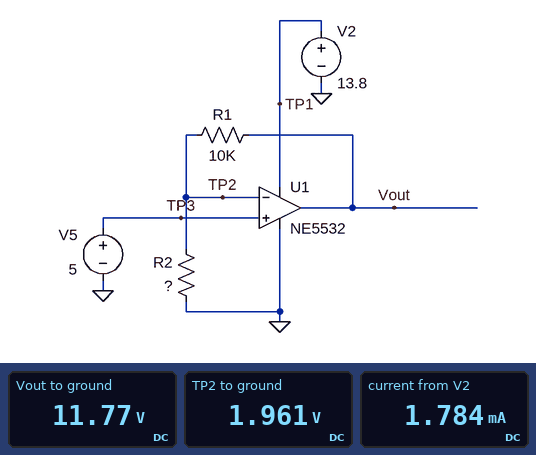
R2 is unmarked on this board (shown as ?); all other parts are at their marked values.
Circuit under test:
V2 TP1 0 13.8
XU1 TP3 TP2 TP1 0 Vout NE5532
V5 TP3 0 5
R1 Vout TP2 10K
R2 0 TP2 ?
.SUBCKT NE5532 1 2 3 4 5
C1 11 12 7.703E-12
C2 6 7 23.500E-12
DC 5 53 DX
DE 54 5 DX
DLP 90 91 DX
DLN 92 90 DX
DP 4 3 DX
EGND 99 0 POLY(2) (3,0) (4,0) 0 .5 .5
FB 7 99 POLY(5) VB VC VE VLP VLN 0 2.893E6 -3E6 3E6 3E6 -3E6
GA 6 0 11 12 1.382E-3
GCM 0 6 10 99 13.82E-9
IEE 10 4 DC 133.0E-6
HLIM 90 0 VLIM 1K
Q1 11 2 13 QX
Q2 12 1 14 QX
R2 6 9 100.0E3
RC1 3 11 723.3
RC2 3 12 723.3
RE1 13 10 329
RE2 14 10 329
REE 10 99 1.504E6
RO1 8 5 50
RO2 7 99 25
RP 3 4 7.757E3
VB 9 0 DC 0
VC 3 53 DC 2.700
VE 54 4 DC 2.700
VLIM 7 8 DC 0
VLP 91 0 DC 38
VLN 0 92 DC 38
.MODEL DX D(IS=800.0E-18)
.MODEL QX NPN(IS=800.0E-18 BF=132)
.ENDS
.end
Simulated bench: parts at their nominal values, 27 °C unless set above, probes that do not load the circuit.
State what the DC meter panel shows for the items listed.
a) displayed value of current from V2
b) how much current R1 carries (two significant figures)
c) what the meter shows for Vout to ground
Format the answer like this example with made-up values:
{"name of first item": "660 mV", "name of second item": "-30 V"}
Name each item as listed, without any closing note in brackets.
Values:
{"displayed value of current from V2": "1.784 mA", "how much current R1 carries": "980 µA", "what the meter shows for Vout to ground": "11.77 V"}
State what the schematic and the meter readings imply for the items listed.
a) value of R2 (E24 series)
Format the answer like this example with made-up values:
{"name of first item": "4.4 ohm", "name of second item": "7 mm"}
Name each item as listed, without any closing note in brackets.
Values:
{"value of R2": "2 kΩ"}
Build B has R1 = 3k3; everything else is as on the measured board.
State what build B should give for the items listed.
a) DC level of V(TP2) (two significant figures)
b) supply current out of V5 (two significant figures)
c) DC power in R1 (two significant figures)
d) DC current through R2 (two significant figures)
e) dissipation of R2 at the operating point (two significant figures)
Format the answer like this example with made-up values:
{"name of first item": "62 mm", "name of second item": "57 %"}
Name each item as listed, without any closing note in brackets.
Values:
{"DC level of V(TP2)": "4.4 V", "supply current out of V5": "990 nA", "DC power in R1": "16 mW", "DC current through R2": "2.2 mA", "dissipation of R2 at the operating point": "9.9 mW"}
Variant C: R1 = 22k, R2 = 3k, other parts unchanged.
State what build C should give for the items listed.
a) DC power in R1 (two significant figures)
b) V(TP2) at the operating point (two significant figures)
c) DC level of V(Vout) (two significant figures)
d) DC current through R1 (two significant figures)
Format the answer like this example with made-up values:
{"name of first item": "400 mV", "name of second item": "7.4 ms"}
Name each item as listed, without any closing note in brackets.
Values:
{"DC power in R1": "4.9 mW", "V(TP2) at the operating point": "1.4 V", "DC level of V(Vout)": "12 V", "DC current through R1": "470 µA"}
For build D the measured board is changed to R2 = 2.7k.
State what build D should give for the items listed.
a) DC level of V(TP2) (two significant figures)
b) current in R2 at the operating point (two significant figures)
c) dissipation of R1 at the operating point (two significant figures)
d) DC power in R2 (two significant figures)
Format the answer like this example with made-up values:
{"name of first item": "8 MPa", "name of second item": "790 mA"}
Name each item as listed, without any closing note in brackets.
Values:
{"DC level of V(TP2)": "2.5 V", "current in R2 at the operating point": "930 µA", "dissipation of R1 at the operating point": "8.6 mW", "DC power in R2": "2.3 mW"}
